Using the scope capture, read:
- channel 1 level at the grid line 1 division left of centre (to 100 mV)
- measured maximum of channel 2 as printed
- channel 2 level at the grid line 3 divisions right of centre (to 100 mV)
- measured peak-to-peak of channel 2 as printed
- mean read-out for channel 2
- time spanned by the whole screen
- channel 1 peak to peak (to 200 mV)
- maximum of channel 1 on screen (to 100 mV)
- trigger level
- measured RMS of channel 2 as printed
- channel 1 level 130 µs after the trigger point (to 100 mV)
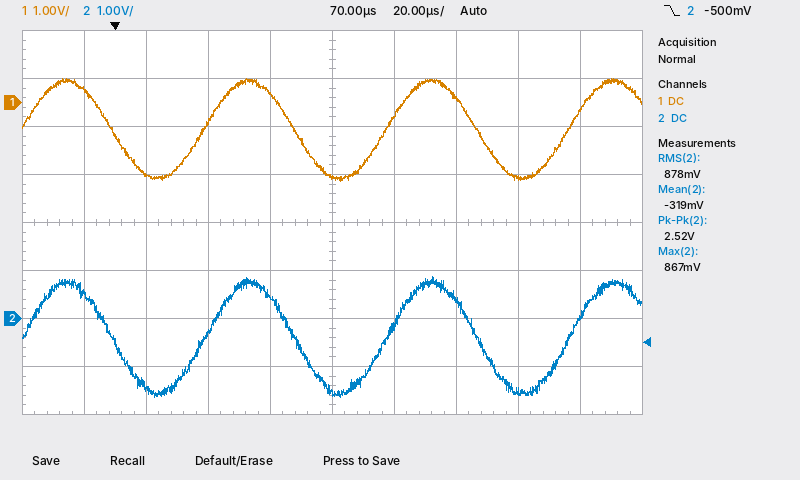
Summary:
200 mV
867 mV
-1.5 V
2.52 V
-319 mV
200 µs
2.2 V
500 mV
-500 mV
878 mV
-1.6 V
